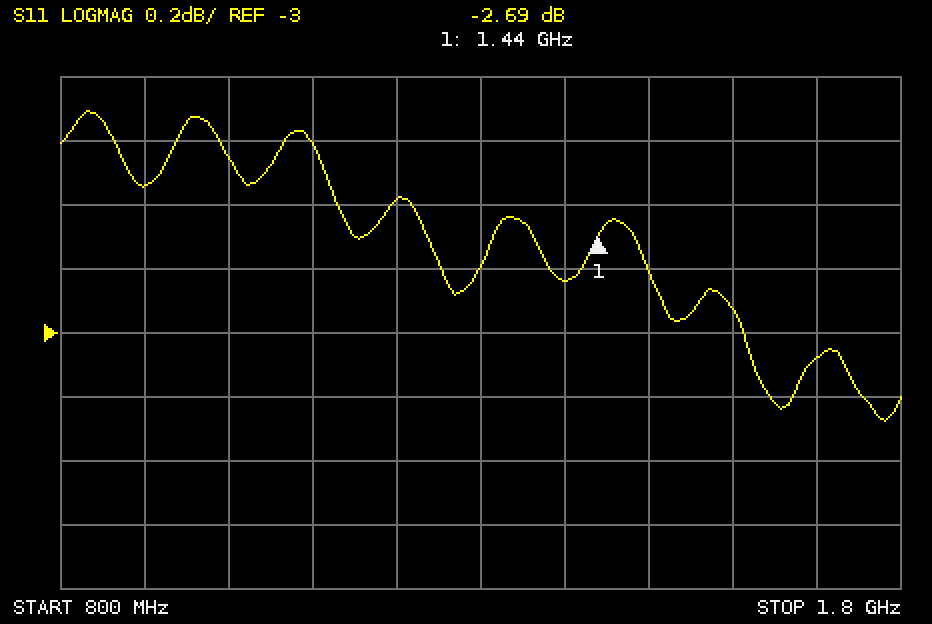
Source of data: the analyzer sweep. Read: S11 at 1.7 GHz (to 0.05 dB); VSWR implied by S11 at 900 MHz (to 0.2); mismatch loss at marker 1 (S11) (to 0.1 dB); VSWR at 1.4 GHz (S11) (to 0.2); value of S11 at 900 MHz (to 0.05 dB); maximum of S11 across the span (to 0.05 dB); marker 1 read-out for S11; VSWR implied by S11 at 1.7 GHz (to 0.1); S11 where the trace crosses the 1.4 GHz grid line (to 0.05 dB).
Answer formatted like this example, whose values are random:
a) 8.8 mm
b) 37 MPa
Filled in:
a) -3.10 dB
b) 6.8
c) 3.4 dB
d) 6.2
e) -2.55 dB
f) -2.30 dB
g) -2.69 dB
h) 5.7
i) -2.85 dB
